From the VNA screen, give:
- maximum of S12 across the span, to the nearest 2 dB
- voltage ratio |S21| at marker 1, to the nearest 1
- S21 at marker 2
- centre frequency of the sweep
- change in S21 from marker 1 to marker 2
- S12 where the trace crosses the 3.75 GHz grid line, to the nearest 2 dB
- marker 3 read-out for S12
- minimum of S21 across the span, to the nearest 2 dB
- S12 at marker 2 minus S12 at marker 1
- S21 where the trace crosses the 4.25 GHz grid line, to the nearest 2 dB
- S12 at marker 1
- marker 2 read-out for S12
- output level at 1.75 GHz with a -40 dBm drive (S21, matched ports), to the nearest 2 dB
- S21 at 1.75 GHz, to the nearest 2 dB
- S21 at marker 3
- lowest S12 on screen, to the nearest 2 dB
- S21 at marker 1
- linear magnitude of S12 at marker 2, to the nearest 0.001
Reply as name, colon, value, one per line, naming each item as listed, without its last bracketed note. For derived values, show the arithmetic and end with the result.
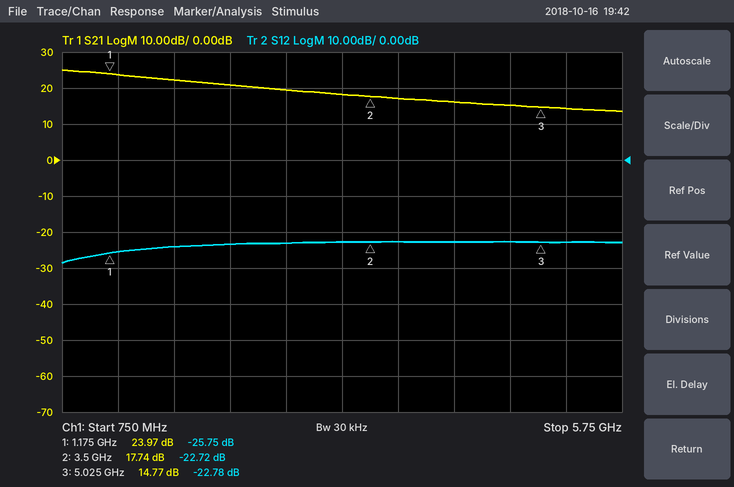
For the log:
maximum of S12 across the span, to the nearest 2 dB: -22 dB
voltage ratio |S21| at marker 1, to the nearest 1: 10^(23.97/20) ≈ 16
S21 at marker 2: 17.74 dB
centre frequency of the sweep: 3.25 GHz
change in S21 from marker 1 to marker 2: 17.74 − (23.97) = -6.23 dB
S12 where the trace crosses the 3.75 GHz grid line, to the nearest 2 dB: -22 dB
marker 3 read-out for S12: -22.78 dB
minimum of S21 across the span, to the nearest 2 dB: 14 dB
S12 at marker 2 minus S12 at marker 1: -22.72 − (-25.75) = 3.03 dB
S21 where the trace crosses the 4.25 GHz grid line, to the nearest 2 dB: 16 dB
S12 at marker 1: -25.75 dB
marker 2 read-out for S12: -22.72 dB
output level at 1.75 GHz with a -40 dBm drive (S21, matched ports), to the nearest 2 dB: -40 dBm + (22 dB) = -18 dBm
S21 at 1.75 GHz, to the nearest 2 dB: 22 dB
S21 at marker 3: 14.77 dB
lowest S12 on screen, to the nearest 2 dB: -28 dB
S21 at marker 1: 23.97 dB
linear magnitude of S12 at marker 2, to the nearest 0.001: 10^(-22.72/20) ≈ 0.073
